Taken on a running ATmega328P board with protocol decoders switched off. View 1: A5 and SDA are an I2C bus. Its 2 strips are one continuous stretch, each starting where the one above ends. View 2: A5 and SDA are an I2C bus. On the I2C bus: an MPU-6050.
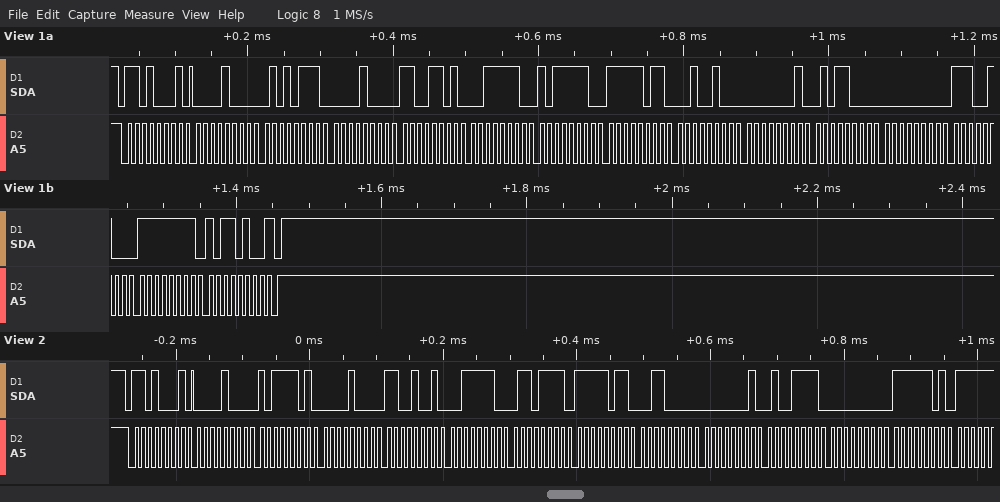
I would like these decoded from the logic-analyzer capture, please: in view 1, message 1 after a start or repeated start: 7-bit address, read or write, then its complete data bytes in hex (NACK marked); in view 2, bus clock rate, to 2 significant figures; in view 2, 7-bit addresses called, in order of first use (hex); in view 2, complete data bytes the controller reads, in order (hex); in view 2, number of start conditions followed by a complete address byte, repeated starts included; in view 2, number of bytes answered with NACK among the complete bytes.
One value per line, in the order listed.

0x68 read: 08 57 08 CD 3E BE FB 24 01 58 00 E4 FF B4 NACK
100 kHz
0x68
08 BD 08 C9 3E 6F FB 30 01 4F 00 FD
1
0
